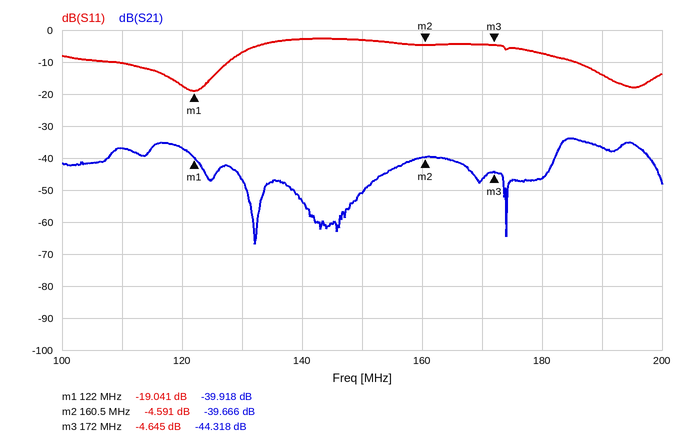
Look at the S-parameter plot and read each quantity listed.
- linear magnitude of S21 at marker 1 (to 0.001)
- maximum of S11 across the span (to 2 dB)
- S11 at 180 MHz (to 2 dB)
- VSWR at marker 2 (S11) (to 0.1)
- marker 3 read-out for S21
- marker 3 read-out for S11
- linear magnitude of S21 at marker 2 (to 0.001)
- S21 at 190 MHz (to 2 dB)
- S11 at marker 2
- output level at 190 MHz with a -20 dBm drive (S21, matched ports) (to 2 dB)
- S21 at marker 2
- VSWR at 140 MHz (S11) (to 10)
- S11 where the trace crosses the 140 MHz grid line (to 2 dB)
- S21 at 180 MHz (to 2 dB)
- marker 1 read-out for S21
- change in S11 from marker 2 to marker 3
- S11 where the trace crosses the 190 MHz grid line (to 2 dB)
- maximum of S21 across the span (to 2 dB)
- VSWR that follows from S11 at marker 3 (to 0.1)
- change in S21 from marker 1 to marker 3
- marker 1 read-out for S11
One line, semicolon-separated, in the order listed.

0.010; -2 dB; -8 dB; 3.9; -44.318 dB; -4.645 dB; 0.010; -36 dB; -4.591 dB; -56 dBm; -39.666 dB; 10; -2 dB; -46 dB; -39.918 dB; -0.054 dB; -14 dB; -34 dB; 3.8; -4.400 dB; -19.041 dB
